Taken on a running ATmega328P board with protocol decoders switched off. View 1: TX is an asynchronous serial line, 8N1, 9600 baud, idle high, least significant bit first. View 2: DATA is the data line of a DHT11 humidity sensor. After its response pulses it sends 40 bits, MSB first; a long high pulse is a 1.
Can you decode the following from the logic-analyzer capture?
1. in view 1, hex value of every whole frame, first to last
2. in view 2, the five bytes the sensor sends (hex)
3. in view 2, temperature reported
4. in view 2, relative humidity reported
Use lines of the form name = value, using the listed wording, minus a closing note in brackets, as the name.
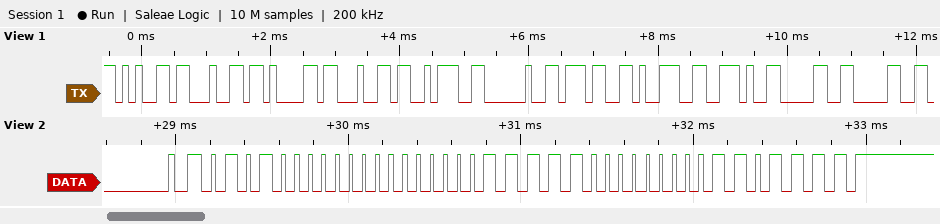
in view 1, hex value of every whole frame, first to last = 65 64 61 64 3A 20 37 39 2E 30 30
in view 2, the five bytes the sensor sends = 50 00 1F 00 6F
in view 2, temperature reported = 31.0 °C
in view 2, relative humidity reported = 80 %
